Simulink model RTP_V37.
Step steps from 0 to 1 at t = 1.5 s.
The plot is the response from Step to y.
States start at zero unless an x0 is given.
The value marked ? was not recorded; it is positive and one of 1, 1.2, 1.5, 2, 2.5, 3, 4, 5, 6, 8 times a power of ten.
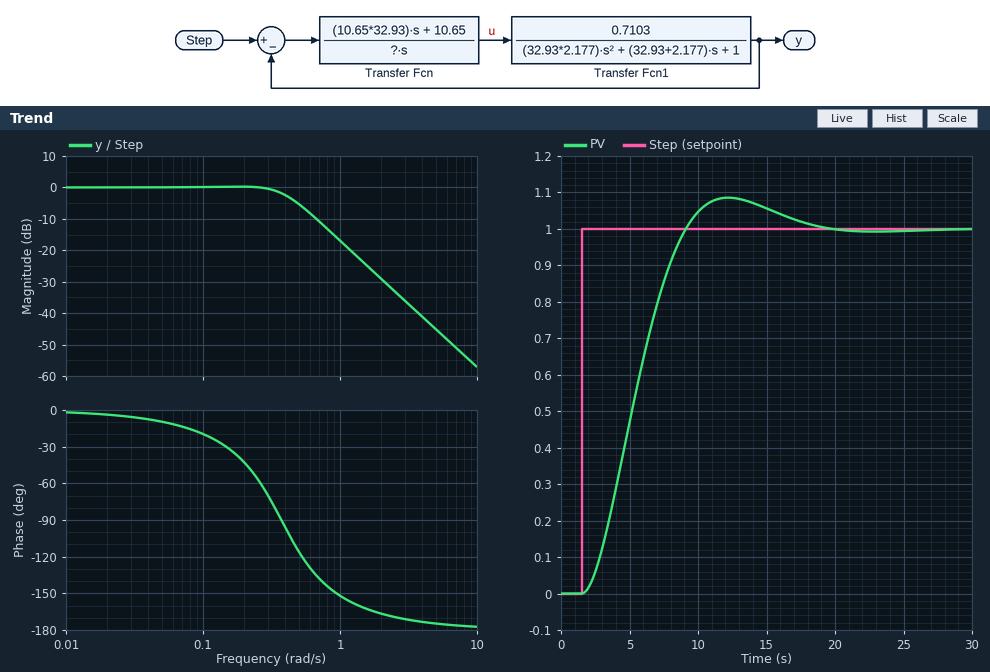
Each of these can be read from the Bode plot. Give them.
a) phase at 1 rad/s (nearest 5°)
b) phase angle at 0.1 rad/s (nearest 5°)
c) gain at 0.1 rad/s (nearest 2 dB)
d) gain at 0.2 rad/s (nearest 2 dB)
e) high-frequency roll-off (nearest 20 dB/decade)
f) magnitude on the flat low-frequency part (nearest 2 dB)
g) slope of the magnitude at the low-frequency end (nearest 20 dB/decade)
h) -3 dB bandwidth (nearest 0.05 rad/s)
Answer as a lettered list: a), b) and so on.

a) -150°
b) -20°
c) 0 dB
d) 0 dB
e) -40 dB/decade
f) 0 dB
g) 0 dB/decade
h) 0.40 rad/s
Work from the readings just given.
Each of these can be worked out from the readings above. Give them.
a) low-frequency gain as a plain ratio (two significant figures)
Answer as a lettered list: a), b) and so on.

a) 1.0
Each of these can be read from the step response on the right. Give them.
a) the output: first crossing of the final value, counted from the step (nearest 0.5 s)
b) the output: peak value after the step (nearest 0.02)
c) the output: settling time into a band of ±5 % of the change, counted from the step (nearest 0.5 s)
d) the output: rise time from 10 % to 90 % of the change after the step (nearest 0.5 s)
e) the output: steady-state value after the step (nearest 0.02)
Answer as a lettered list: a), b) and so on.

a) 7.5 s
b) 1.08
c) 14.0 s
d) 5.0 s
e) 1.00
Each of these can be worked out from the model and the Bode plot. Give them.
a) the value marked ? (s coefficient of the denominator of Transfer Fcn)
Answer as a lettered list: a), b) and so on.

a) 25
